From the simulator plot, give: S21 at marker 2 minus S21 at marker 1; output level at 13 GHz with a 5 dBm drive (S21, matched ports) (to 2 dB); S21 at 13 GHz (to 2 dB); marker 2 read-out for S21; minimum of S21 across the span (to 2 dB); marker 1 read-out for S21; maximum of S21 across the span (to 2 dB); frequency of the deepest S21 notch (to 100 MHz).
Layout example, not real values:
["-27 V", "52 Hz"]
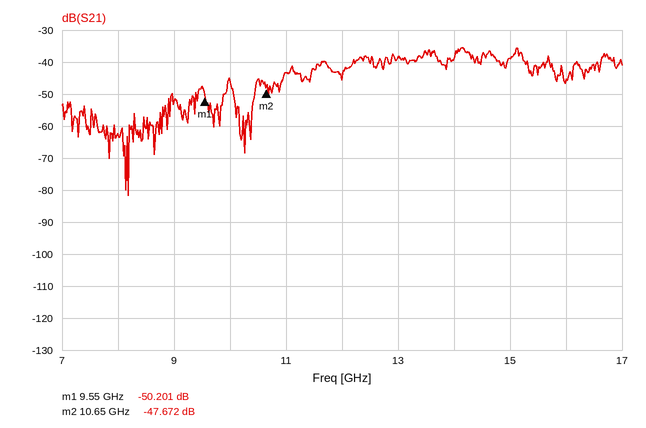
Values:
["2.529 dB", "-34 dBm", "-38 dB", "-47.672 dB", "-82 dB", "-50.201 dB", "-36 dB", "8.2 GHz"]
